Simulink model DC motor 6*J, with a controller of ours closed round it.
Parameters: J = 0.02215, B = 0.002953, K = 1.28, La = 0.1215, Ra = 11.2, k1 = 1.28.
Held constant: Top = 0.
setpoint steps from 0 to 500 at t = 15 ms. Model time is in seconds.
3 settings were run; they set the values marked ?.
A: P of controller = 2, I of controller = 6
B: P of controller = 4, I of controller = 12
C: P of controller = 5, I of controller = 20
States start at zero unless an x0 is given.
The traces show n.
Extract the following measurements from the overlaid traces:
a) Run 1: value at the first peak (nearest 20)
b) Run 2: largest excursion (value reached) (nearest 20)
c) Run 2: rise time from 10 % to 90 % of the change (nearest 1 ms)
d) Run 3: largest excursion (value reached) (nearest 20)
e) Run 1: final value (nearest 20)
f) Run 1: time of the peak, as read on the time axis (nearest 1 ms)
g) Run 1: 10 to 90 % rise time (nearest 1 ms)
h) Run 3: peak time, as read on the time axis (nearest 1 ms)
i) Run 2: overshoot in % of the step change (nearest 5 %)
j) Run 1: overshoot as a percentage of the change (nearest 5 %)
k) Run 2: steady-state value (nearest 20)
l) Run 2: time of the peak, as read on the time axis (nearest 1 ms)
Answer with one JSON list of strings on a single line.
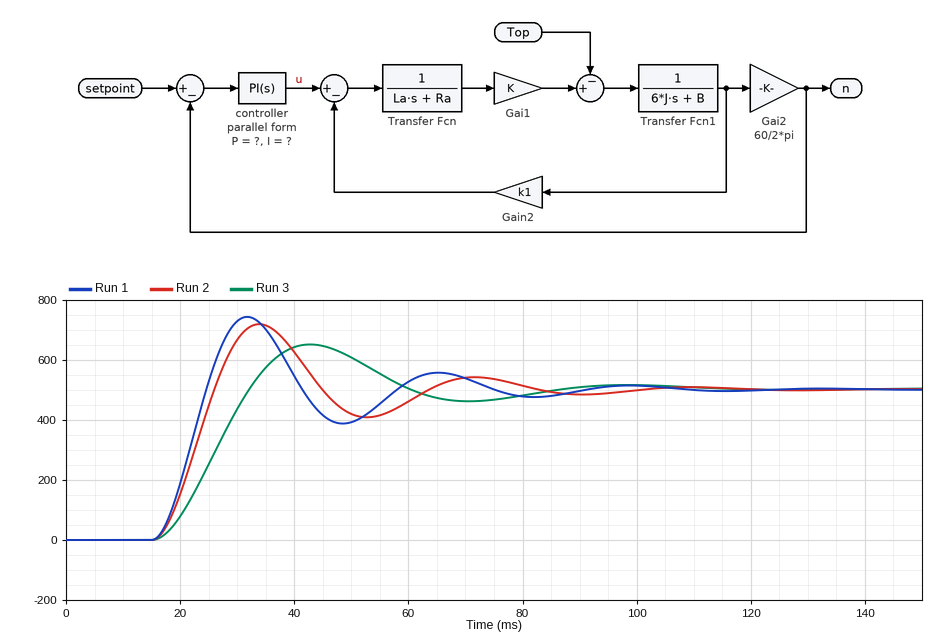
["740", "720", "7 ms", "660", "500", "32 ms", "6 ms", "43 ms", "45 %", "50 %", "500", "34 ms"]
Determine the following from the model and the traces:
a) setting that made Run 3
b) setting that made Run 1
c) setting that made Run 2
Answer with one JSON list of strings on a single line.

["A", "C", "B"]
